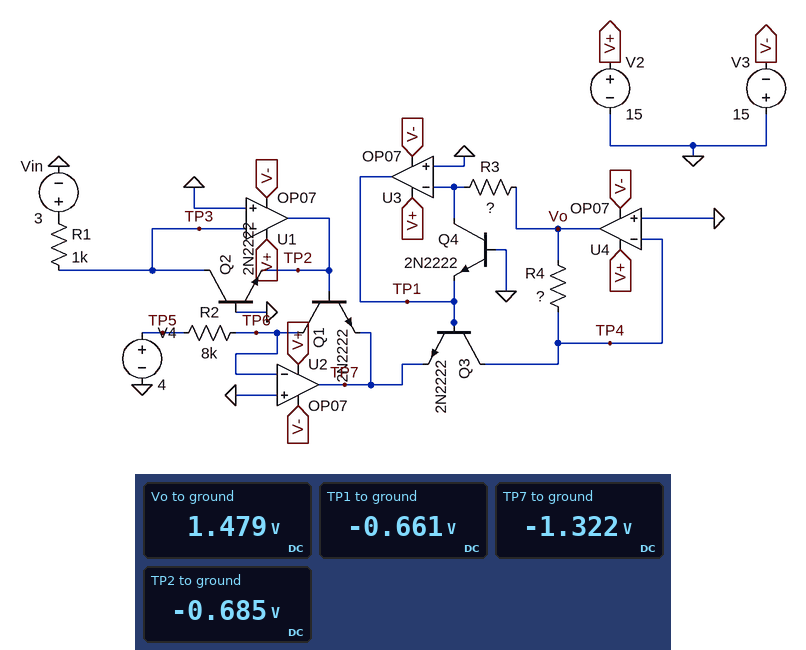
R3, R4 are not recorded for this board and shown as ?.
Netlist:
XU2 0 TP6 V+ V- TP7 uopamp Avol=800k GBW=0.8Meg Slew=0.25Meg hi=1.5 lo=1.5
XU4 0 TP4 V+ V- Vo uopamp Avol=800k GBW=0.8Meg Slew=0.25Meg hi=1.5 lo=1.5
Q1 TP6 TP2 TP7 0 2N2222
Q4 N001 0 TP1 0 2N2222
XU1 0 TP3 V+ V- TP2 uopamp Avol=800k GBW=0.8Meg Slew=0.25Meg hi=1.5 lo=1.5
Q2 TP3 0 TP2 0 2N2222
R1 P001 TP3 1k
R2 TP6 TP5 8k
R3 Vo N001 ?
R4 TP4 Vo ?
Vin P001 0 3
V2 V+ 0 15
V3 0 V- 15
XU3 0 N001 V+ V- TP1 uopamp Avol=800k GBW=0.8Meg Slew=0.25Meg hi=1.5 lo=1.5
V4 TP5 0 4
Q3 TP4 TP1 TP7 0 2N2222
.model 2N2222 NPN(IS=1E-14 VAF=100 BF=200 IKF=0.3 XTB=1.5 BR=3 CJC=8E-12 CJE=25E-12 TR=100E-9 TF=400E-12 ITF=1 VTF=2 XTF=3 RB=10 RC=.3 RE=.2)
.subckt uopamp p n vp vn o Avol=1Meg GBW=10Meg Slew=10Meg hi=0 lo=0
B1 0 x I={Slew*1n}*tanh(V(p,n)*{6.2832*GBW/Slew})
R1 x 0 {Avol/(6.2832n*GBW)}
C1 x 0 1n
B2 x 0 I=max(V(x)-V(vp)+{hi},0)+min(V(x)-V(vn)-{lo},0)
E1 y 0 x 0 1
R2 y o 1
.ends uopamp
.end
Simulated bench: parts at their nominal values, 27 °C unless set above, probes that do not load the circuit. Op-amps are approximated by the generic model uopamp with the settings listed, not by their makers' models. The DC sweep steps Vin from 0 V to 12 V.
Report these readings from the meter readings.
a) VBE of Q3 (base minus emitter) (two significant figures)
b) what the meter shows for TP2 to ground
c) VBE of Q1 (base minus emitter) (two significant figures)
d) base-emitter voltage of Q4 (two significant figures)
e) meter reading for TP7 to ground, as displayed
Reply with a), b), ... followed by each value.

a) 660 mV
b) -0.685 V
c) 640 mV
d) 660 mV
e) -1.322 V
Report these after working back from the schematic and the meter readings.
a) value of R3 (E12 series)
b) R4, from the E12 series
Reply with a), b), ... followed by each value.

a) 1.2 kΩ
b) 1.2 kΩ
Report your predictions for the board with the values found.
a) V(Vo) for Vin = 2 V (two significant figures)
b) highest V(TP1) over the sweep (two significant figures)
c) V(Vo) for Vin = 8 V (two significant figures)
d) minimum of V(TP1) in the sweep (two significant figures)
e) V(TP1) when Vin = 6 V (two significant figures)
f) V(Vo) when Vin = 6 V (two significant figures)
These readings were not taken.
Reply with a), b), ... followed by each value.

a) 1.2 V
b) -320 mV
c) 2.5 V
d) -680 mV
e) -670 mV
f) 2.1 V
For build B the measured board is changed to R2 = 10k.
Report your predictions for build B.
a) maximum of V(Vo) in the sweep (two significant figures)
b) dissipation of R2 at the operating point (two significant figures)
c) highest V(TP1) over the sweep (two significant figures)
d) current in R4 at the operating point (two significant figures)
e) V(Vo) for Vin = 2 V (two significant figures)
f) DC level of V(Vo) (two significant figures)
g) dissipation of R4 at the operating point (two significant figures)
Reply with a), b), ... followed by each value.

a) 2.8 V
b) 1.6 mW
c) -310 mV
d) 1.1 mA
e) 1.1 V
f) 1.3 V
g) 1.5 mW
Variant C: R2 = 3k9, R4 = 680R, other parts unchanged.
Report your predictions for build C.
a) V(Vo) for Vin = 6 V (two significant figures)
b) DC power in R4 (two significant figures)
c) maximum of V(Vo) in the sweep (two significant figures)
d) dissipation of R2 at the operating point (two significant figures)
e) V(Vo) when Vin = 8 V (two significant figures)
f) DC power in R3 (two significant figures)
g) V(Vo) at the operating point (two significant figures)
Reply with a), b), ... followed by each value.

a) 2.3 V
b) 3.7 mW
c) 3.3 V
d) 4.1 mW
e) 2.6 V
f) 2.1 mW
g) 1.6 V
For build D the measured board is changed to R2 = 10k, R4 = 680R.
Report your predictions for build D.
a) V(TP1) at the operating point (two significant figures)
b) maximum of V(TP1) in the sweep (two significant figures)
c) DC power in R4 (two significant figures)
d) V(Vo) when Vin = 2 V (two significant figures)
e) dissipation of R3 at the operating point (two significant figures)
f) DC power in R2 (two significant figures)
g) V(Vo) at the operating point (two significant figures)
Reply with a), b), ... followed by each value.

a) -650 mV
b) -310 mV
c) 1.5 mW
d) 810 mV
e) 830 µW
f) 1.6 mW
g) 1.0 V
